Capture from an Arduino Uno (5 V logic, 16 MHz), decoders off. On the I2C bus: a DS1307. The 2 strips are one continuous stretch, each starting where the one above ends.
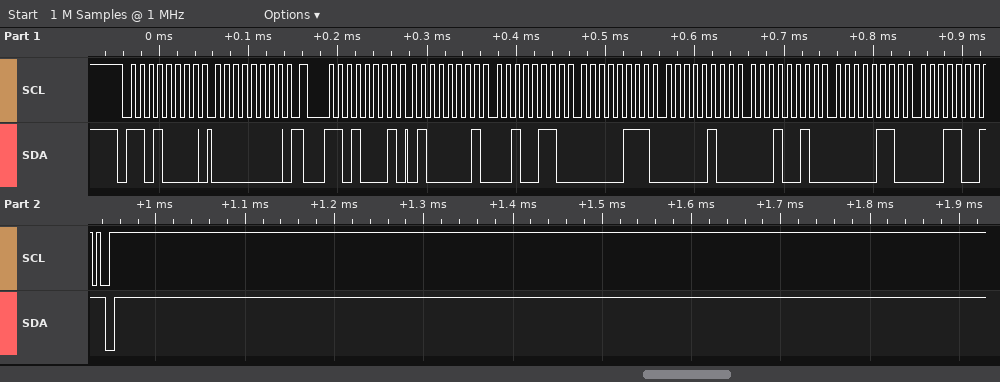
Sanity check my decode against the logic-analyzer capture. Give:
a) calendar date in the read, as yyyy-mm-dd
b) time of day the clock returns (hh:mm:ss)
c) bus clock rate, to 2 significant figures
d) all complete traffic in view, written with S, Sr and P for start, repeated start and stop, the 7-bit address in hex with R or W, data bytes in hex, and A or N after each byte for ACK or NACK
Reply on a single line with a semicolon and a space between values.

2019-06-12; 07:26:41; 100 kHz; S 68W A 00 A Sr 68R A 41 A 26 A 07 A 04 A 12 A 06 A 19 N P
